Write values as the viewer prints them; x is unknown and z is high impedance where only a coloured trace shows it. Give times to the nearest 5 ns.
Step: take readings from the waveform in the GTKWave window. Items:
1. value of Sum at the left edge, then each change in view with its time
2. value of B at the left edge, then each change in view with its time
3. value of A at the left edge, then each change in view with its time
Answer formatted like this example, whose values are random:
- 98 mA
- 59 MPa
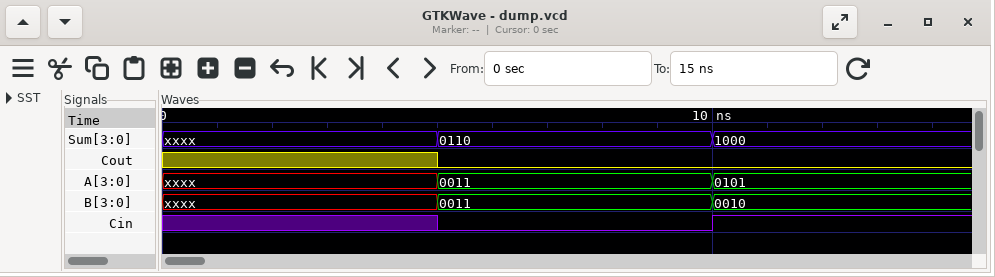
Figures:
- xxxx, 0110 at 5 ns, 1000 at 10 ns
- xxxx, 0011 at 5 ns, 0010 at 10 ns
- xxxx, 0011 at 5 ns, 0101 at 10 ns
